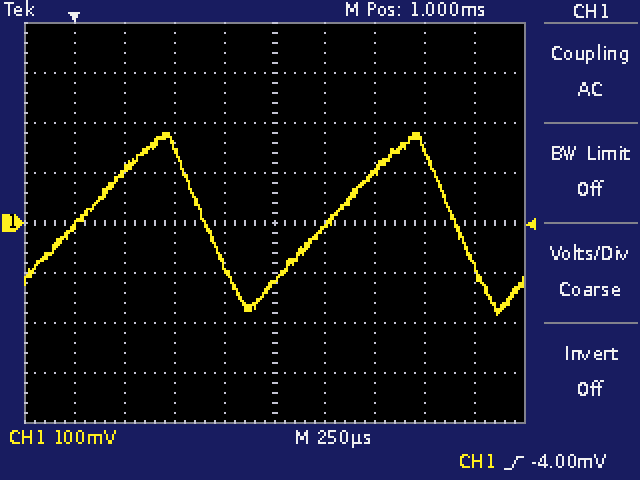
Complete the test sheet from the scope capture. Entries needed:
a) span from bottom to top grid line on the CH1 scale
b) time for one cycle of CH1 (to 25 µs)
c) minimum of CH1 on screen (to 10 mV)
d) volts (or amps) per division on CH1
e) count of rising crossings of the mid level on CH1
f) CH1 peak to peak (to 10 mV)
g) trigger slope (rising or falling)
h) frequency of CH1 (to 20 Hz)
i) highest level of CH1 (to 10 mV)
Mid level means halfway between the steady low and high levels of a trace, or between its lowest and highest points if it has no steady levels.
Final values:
800 mV
1.250 ms
-180 mV
100 mV
2
360 mV
rising
800 Hz
180 mV
